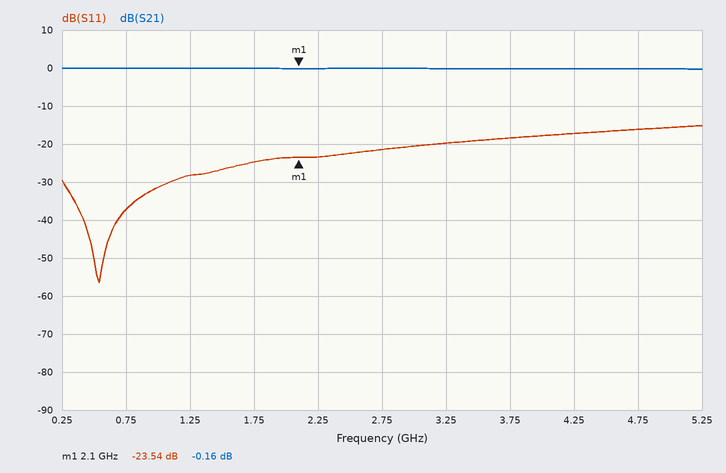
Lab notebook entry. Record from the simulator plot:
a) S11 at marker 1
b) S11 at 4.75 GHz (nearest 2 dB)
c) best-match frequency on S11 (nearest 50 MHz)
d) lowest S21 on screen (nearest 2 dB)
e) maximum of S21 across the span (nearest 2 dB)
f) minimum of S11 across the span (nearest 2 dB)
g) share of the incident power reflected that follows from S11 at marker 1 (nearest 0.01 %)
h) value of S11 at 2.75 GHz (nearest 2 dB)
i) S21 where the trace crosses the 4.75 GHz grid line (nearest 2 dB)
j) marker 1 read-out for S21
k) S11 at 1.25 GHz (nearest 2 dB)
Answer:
-23.54 dB
-16 dB
550 MHz
0 dB
0 dB
-56 dB
0.44 %
-22 dB
0 dB
-0.16 dB
-28 dB
